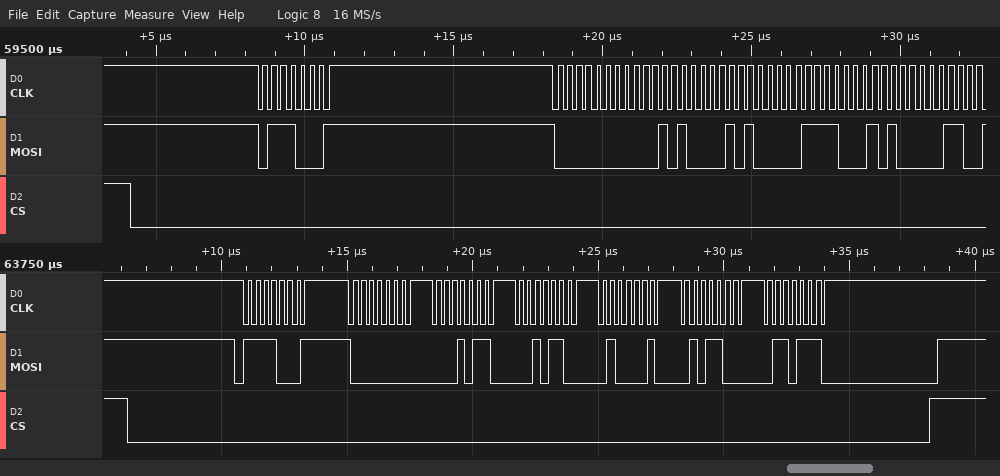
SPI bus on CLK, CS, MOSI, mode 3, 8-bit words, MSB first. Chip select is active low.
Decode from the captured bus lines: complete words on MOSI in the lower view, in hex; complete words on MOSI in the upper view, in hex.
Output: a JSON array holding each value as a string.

["F1, 00, 16, 2C, 42, 58, 6E", "71, 00, 14, 28, 3C, 50"]
